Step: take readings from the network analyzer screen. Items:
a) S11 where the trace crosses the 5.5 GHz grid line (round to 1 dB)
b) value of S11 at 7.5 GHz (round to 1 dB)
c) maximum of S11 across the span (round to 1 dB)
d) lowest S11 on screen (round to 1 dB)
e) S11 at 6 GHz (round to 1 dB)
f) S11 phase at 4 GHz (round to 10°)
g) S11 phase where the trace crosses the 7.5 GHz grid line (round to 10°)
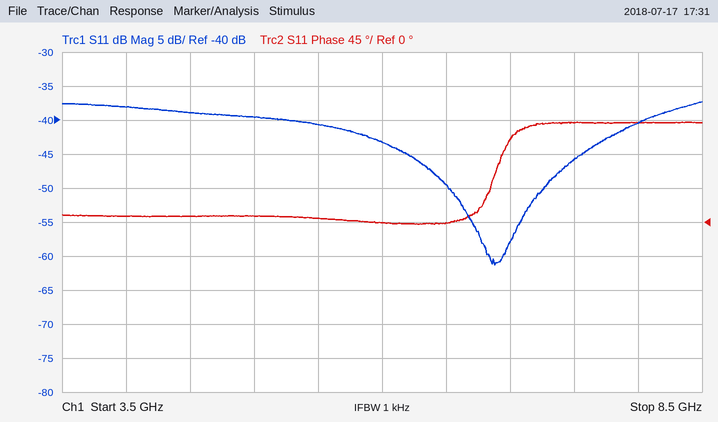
-41 dB
-46 dB
-37 dB
-61 dB
-43 dB
10°
130°
